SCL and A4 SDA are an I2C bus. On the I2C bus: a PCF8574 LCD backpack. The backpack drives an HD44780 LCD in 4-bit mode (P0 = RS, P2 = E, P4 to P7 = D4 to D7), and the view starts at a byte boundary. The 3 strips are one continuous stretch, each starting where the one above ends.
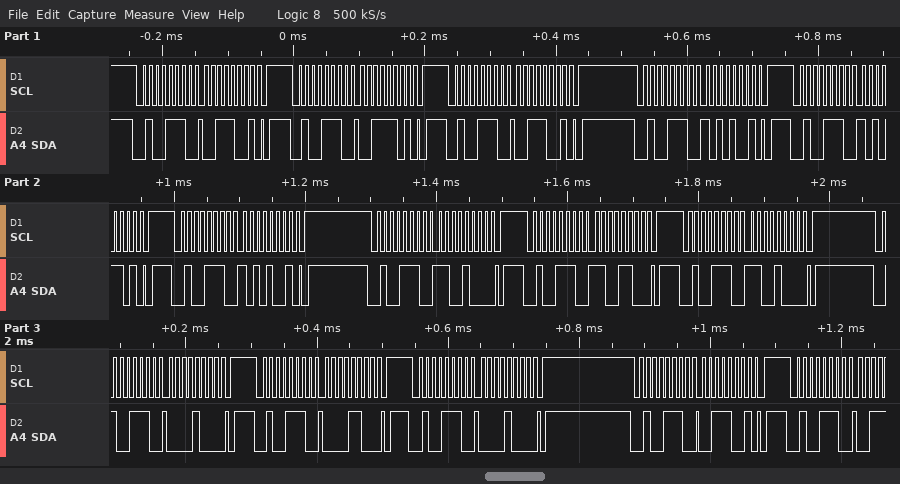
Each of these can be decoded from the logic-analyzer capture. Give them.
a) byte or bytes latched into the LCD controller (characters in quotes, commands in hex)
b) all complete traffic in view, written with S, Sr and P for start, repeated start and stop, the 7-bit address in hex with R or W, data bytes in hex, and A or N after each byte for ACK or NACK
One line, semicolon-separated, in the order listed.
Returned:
':' 0xC0; S 27W A 39 A P S 27W A 3D A P S 27W A 39 A P S 27W A A9 A P S 27W A AD A P S 27W A A9 A P S 27W A C8 A P S 27W A CC A P S 27W A C8 A P S 27W A 08 A P S 27W A 0C A P S 27W A 08 A P S 27W A 39 A P S 27W A
